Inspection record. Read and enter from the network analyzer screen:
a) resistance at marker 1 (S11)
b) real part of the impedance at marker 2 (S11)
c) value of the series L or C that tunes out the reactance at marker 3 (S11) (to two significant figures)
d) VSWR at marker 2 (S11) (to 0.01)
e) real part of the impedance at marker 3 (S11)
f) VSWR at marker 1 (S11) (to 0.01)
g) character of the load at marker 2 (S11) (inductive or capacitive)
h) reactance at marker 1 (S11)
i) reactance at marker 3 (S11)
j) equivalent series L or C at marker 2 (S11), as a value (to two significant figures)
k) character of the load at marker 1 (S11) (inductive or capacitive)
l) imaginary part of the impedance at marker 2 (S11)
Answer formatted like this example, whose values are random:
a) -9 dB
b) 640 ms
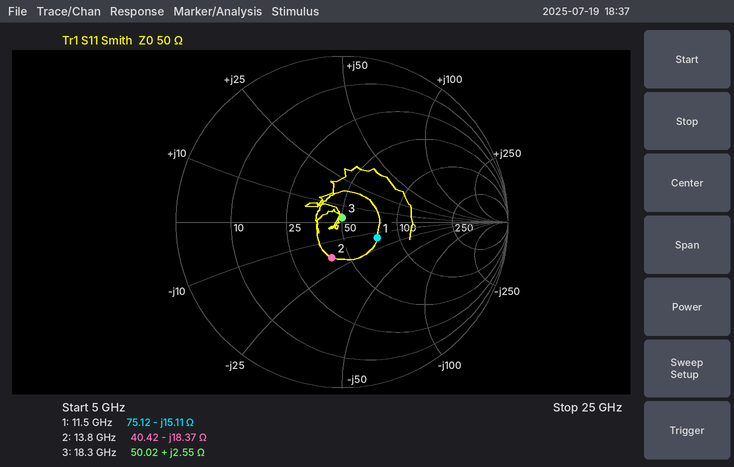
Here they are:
a) 75.12 Ω
b) 40.42 Ω
c) 3.4 pF
d) 1.58
e) 50.02 Ω
f) 1.61
g) capacitive
h) -15.11 Ω
i) +2.55 Ω
j) 630 fF
k) capacitive
l) -18.37 Ω
